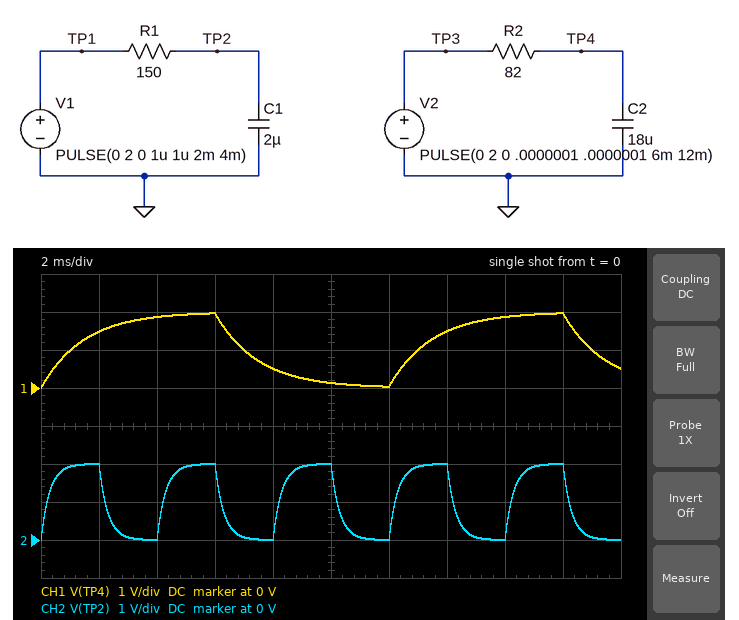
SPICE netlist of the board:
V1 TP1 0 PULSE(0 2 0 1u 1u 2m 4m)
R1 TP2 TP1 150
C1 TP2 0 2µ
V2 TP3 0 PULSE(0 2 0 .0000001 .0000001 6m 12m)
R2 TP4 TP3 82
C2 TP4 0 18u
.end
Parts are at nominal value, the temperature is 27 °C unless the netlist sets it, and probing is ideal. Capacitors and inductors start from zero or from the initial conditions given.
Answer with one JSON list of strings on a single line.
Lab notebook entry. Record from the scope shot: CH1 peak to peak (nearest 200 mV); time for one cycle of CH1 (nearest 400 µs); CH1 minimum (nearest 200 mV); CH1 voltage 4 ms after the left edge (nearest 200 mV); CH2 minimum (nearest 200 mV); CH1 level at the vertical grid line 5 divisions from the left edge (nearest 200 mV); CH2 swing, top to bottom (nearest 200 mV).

["2.0 V", "12.0 ms", "0 V", "1.8 V", "0 V", "200 mV", "2.0 V"]
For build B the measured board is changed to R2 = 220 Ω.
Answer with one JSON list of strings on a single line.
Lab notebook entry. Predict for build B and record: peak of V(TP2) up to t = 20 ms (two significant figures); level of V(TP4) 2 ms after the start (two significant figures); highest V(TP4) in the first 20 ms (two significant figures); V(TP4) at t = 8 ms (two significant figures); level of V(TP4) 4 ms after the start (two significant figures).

["2.0 V", "790 mV", "1.6 V", "940 mV", "1.3 V"]
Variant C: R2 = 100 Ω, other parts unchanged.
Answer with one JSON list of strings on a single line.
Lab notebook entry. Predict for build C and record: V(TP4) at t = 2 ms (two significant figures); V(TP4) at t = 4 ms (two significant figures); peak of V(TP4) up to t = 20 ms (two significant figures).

["1.3 V", "1.8 V", "1.9 V"]
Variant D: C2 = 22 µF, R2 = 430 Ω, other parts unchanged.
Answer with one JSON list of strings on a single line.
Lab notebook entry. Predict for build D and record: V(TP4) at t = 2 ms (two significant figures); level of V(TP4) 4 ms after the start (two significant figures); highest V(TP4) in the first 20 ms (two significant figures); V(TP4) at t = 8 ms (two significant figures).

["380 mV", "690 mV", "1.2 V", "760 mV"]
